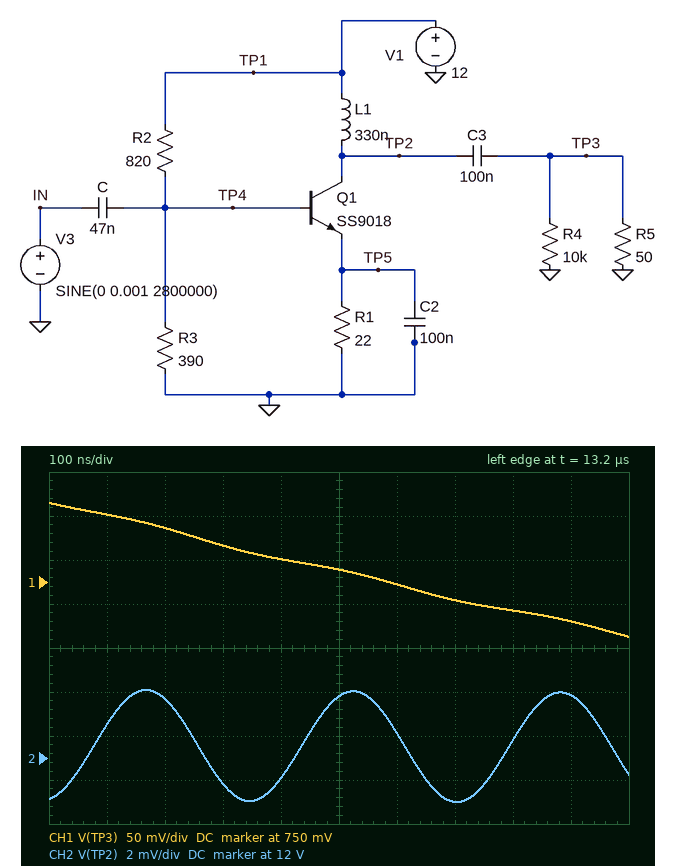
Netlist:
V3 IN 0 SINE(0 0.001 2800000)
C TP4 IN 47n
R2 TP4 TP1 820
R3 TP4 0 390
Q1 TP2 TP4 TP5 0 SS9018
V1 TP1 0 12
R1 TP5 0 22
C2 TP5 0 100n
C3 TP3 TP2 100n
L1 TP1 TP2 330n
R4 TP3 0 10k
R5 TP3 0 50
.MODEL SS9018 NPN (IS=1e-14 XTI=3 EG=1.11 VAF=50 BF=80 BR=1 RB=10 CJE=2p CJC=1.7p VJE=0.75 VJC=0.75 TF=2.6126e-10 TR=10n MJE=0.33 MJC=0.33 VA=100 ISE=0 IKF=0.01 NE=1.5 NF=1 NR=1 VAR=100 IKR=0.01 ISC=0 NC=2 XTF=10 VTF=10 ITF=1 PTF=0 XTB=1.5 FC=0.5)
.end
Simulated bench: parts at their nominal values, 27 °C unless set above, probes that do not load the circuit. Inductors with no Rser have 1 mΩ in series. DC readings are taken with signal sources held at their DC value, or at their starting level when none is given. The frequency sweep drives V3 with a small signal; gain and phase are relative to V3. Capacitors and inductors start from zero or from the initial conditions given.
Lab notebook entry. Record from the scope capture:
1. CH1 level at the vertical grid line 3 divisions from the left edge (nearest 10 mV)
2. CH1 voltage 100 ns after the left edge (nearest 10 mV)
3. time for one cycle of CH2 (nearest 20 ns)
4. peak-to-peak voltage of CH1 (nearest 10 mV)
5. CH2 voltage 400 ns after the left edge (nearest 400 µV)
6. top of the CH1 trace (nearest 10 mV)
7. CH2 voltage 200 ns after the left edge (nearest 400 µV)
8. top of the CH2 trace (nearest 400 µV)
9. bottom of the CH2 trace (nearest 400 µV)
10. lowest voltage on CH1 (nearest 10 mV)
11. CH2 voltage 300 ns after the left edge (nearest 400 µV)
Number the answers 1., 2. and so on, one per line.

1. 790 mV
2. 830 mV
3. 360 ns
4. 150 mV
5. 11.9992 V
6. 840 mV
7. 12.0028 V
8. 12.0032 V
9. 11.9980 V
10. 690 mV
11. 11.9988 V
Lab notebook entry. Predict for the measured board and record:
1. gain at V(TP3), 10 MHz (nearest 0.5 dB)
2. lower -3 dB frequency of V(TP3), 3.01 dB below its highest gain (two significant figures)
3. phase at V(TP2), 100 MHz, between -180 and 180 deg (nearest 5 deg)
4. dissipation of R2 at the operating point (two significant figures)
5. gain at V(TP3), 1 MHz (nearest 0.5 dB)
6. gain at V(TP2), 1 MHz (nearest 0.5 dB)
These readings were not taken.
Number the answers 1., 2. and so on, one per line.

1. 18.5 dB
2. 13 MHz
3. 125 deg
4. 110 mW
5. -4.0 dB
6. -4.0 dB
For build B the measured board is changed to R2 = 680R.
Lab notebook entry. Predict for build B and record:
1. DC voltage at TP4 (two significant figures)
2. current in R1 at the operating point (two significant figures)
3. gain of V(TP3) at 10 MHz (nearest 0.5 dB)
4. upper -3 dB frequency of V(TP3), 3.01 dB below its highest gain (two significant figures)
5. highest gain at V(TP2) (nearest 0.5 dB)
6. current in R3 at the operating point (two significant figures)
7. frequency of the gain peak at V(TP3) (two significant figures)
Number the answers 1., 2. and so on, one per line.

1. 2.7 V
2. 82 mA
3. 18.0 dB
4. 75 MHz
5. 22.5 dB
6. 6.9 mA
7. 31 MHz
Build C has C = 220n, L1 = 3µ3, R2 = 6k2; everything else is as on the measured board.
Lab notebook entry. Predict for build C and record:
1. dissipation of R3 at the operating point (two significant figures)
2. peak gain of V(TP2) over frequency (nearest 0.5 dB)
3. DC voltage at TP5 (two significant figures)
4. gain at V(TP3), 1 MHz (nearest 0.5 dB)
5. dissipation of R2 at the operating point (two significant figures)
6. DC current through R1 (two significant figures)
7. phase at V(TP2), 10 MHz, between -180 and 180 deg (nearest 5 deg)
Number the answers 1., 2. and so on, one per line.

1. 1.3 mW
2. 8.5 dB
3. 35 mV
4. 0 dB
5. 21 mW
6. 1.6 mA
7. -165 deg
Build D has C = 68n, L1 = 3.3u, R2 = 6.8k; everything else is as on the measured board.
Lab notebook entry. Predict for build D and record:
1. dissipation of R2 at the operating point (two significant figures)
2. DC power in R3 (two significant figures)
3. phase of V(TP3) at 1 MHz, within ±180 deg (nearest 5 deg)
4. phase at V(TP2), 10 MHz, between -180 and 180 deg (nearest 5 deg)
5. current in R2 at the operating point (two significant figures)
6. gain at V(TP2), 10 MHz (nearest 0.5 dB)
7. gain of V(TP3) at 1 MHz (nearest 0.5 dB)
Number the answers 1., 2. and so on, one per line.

1. 19 mW
2. 1.1 mW
3. -110 deg
4. -165 deg
5. 1.7 mA
6. -0.5 dB
7. -8.5 dB
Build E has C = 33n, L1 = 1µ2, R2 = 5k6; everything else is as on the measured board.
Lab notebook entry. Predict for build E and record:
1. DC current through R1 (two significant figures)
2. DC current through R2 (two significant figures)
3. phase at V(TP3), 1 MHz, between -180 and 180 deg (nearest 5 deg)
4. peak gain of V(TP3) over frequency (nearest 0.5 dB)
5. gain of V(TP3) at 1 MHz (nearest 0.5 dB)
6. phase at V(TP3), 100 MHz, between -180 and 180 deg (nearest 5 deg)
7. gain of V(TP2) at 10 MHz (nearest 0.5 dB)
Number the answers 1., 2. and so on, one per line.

1. 3.3 mA
2. 2.0 mA
3. -85 deg
4. 14.0 dB
5. -2.5 dB
6. 170 deg
7. 12.5 dB
